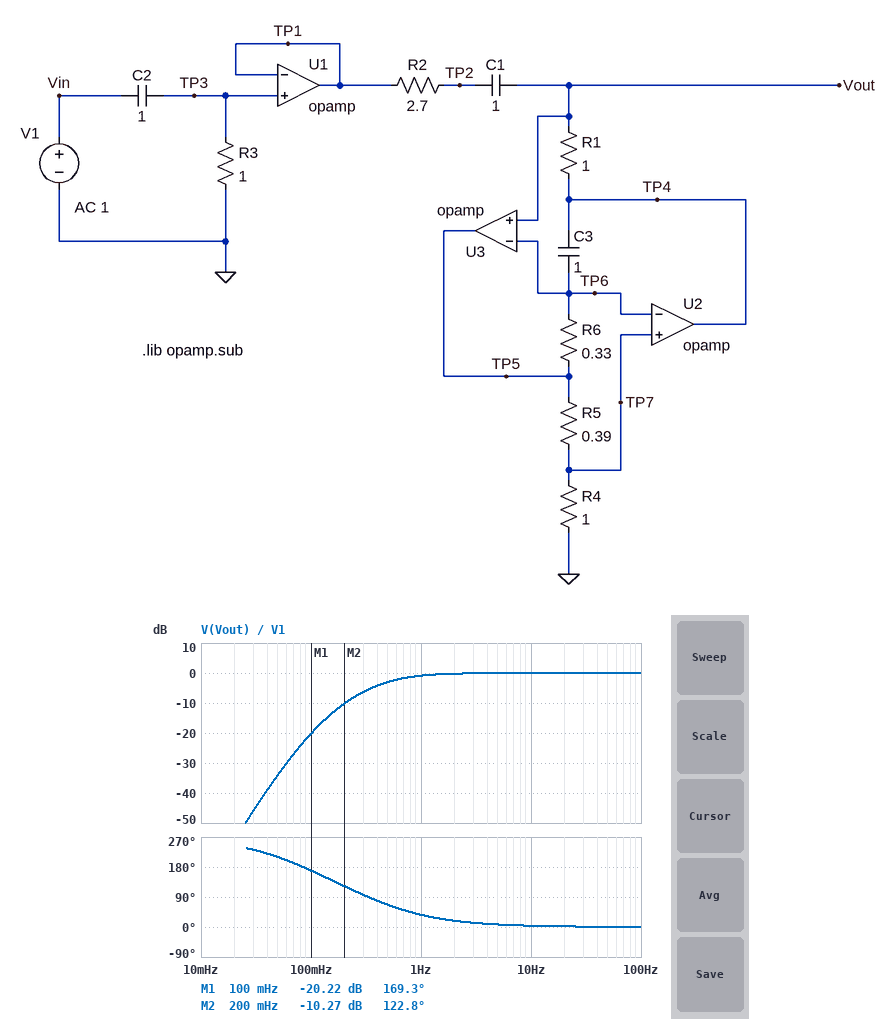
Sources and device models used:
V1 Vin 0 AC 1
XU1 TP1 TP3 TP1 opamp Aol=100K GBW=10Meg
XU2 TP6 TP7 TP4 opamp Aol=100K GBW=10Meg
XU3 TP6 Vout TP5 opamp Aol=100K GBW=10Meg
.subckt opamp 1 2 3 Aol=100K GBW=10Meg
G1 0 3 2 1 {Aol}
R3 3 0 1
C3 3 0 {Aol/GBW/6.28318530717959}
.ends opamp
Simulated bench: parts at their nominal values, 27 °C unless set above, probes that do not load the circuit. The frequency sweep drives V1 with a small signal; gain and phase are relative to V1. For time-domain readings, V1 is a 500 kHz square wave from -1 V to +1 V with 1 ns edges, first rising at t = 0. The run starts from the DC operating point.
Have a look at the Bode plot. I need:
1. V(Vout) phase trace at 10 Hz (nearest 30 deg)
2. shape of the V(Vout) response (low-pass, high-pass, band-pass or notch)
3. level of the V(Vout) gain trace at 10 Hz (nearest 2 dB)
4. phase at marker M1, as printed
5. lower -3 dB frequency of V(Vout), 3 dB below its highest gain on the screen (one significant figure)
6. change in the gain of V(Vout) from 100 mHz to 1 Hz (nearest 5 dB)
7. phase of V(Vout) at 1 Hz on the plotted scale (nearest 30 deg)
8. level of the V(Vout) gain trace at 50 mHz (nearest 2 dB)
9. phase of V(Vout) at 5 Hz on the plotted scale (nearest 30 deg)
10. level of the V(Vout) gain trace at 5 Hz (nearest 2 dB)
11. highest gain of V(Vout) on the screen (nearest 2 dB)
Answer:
0 deg
high-pass
0 dB
169.3 deg
500 mHz
20 dB
30 deg
-34 dB
0 deg
0 dB
0 dB
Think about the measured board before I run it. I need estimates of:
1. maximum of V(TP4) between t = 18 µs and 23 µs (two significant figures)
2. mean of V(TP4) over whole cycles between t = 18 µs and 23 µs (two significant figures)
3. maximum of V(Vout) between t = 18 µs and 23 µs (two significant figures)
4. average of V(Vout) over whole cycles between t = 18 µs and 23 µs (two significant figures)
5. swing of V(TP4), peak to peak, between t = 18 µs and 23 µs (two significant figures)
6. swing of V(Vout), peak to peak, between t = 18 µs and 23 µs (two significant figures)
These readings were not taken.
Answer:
2.0 V
1.0 V
2.0 V
1.0 V
2.0 V
2.0 V
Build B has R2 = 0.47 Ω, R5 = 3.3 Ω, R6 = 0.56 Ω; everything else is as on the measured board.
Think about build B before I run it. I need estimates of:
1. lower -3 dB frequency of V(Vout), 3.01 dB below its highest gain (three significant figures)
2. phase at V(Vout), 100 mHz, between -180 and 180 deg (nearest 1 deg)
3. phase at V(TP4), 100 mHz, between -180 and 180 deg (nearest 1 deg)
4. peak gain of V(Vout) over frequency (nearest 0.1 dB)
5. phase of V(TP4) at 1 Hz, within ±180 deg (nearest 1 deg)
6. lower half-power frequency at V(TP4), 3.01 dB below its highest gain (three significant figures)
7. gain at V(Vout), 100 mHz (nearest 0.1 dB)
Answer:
358 mHz
-140 deg
-56 deg
0.3 dB
80 deg
259 mHz
-28.8 dB
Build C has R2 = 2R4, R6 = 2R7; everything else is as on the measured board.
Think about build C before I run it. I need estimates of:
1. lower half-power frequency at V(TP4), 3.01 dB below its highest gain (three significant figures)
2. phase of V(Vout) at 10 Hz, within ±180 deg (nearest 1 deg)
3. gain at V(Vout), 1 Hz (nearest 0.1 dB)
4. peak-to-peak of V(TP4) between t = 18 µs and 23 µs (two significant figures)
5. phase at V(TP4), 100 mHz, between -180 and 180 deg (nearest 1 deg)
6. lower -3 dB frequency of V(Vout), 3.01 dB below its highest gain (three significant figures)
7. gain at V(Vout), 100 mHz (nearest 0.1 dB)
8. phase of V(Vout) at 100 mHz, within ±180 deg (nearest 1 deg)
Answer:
123 mHz
1 deg
-0.1 dB
2.0 V
112 deg
129 mHz
-4.0 dB
99 deg
